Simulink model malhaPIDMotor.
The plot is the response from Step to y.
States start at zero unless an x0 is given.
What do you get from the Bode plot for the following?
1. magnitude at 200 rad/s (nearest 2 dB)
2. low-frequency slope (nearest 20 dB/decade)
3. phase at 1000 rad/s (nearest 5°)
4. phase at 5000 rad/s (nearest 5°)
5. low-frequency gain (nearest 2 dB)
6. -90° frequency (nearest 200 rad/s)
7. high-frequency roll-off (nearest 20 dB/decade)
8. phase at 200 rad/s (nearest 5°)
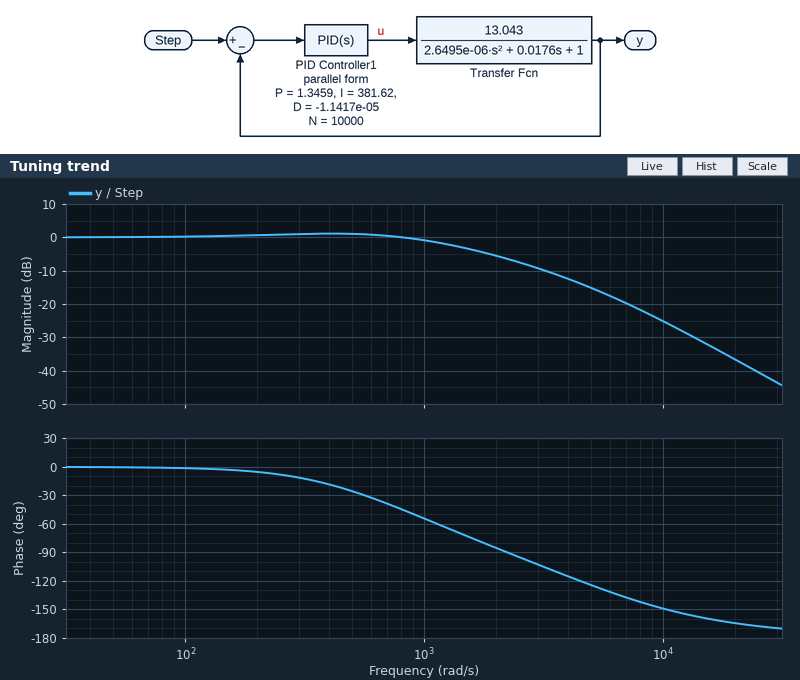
0 dB
0 dB/decade
-55°
-125°
0 dB
2200 rad/s
-40 dB/decade
-5°
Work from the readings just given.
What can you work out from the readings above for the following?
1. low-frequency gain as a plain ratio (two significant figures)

1.0
